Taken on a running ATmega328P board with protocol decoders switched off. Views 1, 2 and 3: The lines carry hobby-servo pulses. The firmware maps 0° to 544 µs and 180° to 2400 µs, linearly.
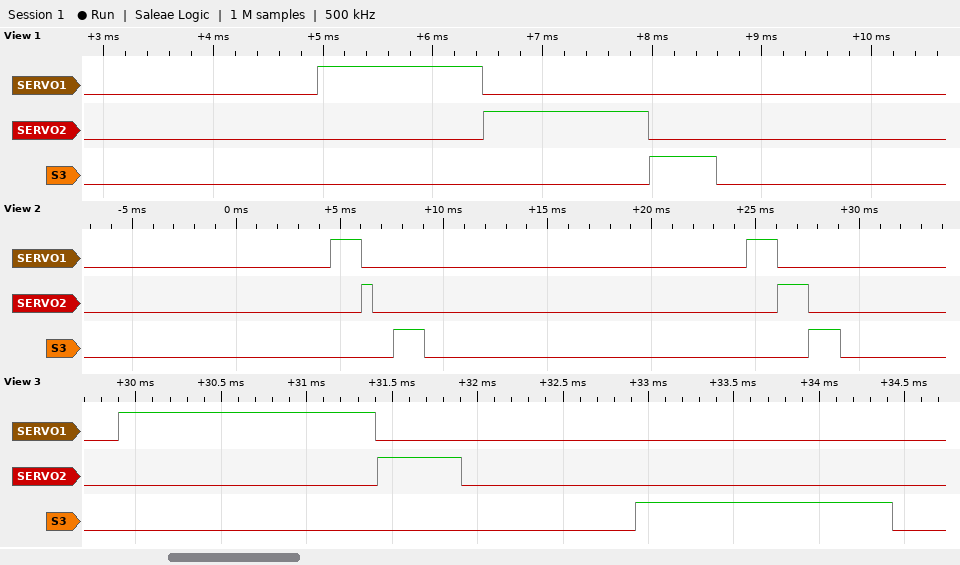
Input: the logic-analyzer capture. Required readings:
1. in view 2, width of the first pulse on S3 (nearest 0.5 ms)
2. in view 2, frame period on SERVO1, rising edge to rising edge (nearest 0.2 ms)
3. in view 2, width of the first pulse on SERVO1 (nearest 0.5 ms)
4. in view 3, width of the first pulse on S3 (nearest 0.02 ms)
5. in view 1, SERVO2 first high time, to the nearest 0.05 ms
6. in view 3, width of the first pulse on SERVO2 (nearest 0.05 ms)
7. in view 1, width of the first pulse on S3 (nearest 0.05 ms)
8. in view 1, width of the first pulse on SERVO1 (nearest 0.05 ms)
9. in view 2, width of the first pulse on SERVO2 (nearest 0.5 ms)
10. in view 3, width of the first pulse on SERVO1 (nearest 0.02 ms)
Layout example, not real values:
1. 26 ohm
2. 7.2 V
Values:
1. 1.5 ms
2. 20.0 ms
3. 1.5 ms
4. 1.50 ms
5. 1.50 ms
6. 0.50 ms
7. 0.60 ms
8. 1.50 ms
9. 0.5 ms
10. 1.50 ms
